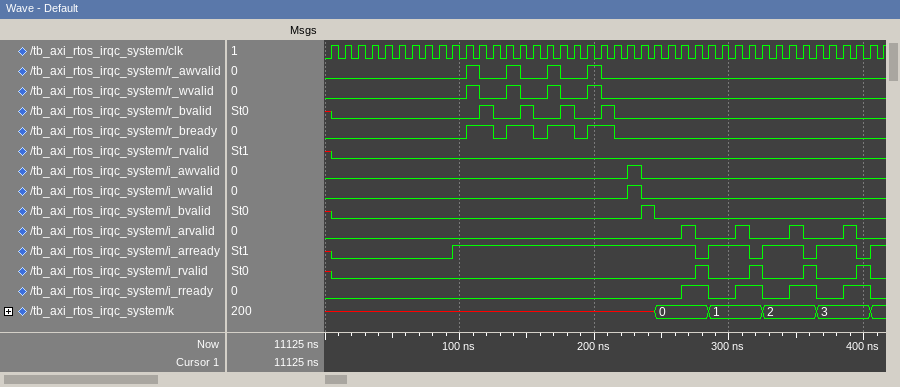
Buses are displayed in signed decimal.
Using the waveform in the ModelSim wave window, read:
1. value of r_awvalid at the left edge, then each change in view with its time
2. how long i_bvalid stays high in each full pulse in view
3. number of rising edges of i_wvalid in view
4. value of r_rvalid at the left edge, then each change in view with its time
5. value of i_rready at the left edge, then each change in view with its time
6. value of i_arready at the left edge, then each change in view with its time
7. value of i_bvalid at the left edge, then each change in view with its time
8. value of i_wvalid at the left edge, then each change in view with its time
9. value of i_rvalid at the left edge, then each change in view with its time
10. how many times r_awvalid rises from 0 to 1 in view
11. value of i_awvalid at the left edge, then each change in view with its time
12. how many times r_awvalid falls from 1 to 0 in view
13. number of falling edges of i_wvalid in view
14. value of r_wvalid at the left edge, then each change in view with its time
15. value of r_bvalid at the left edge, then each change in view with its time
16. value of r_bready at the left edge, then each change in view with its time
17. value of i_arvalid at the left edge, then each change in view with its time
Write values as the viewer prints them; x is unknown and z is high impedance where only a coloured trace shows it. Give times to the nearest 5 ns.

0, 1 at 105 ns, 0 at 115 ns, 1 at 135 ns, 0 at 145 ns, 1 at 165 ns, 0 at 175 ns, 1 at 195 ns, 0 at 205 ns
10 ns
1
x, 0 at 5 ns
0, 1 at 265 ns, 0 at 285 ns, 1 at 305 ns, 0 at 325 ns, 1 at 345 ns, 0 at 365 ns, 1 at 385 ns, 0 at 405 ns
x, 0 at 5 ns, 1 at 95 ns, 0 at 275 ns, 1 at 285 ns, 0 at 315 ns, 1 at 325 ns, 0 at 355 ns, 1 at 365 ns, 0 at 395 ns, 1 at 405 ns
x, 0 at 5 ns, 1 at 235 ns, 0 at 245 ns
0, 1 at 225 ns, 0 at 235 ns
x, 0 at 5 ns, 1 at 275 ns, 0 at 285 ns, 1 at 315 ns, 0 at 325 ns, 1 at 355 ns, 0 at 365 ns, 1 at 395 ns, 0 at 405 ns
4
0, 1 at 225 ns, 0 at 235 ns
4
1
0, 1 at 105 ns, 0 at 115 ns, 1 at 135 ns, 0 at 145 ns, 1 at 165 ns, 0 at 175 ns, 1 at 195 ns, 0 at 205 ns
x, 0 at 5 ns, 1 at 115 ns, 0 at 125 ns, 1 at 145 ns, 0 at 155 ns, 1 at 175 ns, 0 at 185 ns, 1 at 205 ns, 0 at 215 ns
0, 1 at 105 ns, 0 at 125 ns, 1 at 135 ns, 0 at 155 ns, 1 at 165 ns, 0 at 185 ns, 1 at 195 ns, 0 at 215 ns
0, 1 at 265 ns, 0 at 275 ns, 1 at 305 ns, 0 at 315 ns, 1 at 345 ns, 0 at 355 ns, 1 at 385 ns, 0 at 395 ns
